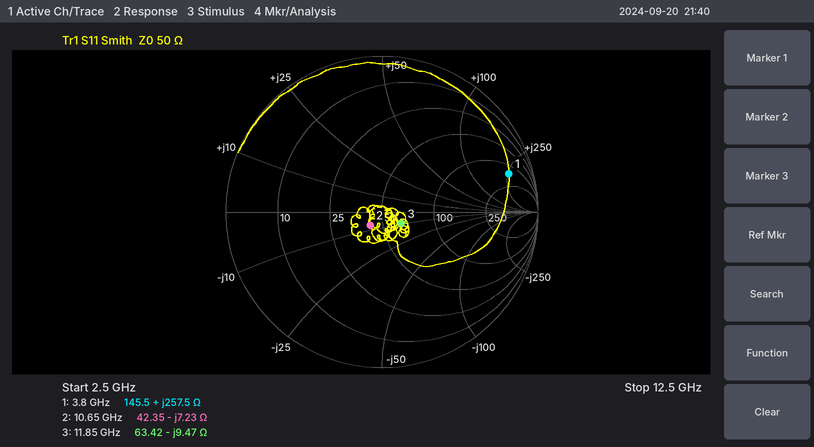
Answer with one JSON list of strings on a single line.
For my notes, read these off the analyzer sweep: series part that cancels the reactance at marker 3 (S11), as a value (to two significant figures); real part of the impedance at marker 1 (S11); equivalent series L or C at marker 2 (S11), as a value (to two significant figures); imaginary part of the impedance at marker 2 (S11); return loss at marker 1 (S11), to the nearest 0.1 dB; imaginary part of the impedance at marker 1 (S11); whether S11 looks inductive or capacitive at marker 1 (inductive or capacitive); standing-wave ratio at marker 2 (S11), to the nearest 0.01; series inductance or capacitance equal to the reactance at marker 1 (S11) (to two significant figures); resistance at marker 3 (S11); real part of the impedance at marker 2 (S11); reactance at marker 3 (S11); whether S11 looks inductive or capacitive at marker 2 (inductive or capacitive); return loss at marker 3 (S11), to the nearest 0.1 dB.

["130 pH", "145.5 Ω", "2.1 pF", "-7.23 Ω", "1.4 dB", "+257.5 Ω", "inductive", "1.26", "11 nH", "63.42 Ω", "42.35 Ω", "-9.47 Ω", "capacitive", "16.8 dB"]
